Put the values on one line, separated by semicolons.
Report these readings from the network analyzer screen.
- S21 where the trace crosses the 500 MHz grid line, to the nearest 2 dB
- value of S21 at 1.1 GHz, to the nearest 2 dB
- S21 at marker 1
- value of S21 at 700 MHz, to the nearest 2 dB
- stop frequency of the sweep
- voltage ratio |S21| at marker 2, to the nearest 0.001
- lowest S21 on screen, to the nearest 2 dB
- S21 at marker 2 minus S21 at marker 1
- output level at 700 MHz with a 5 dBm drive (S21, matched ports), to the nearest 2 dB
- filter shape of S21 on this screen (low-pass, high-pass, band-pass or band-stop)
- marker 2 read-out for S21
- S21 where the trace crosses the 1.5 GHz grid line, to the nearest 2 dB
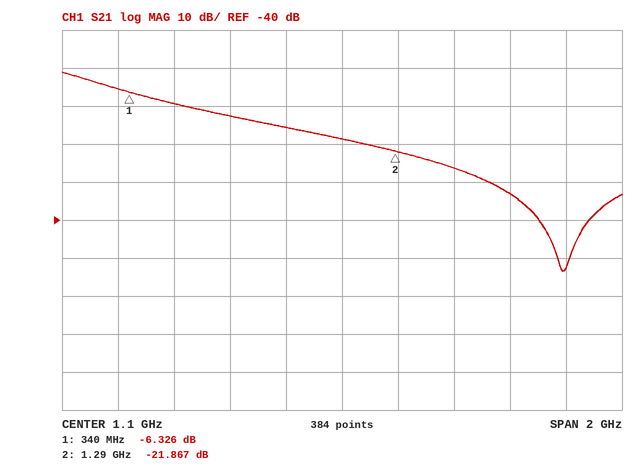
-10 dB; -18 dB; -6.326 dB; -12 dB; 2.1 GHz; 0.081; -54 dB; -15.541 dB; -8 dBm; low-pass; -21.867 dB; -26 dB
